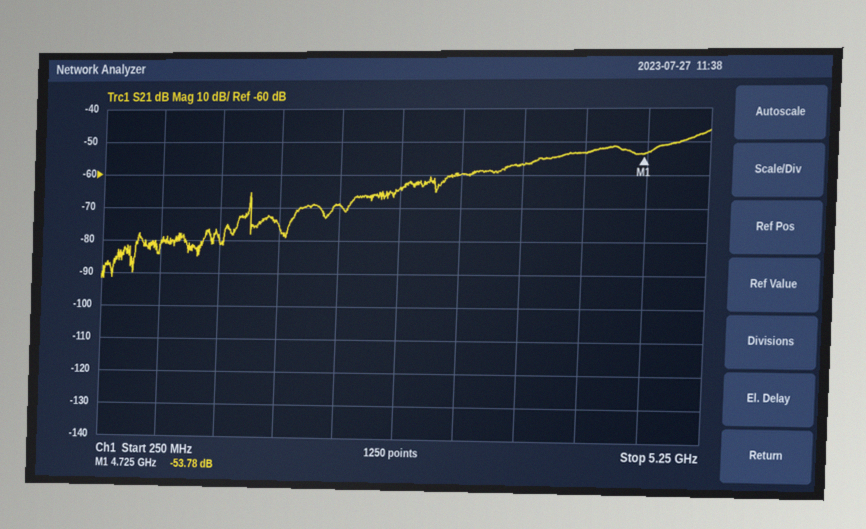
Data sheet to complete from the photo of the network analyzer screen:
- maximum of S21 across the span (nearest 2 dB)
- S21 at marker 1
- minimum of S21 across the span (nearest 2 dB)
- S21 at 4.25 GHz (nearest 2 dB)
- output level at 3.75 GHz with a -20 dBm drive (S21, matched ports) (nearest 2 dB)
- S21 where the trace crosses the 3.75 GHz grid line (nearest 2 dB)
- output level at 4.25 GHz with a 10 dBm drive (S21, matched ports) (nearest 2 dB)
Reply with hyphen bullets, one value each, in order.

- -46 dB
- -53.78 dB
- -92 dB
- -54 dB
- -76 dBm
- -56 dB
- -44 dBm
